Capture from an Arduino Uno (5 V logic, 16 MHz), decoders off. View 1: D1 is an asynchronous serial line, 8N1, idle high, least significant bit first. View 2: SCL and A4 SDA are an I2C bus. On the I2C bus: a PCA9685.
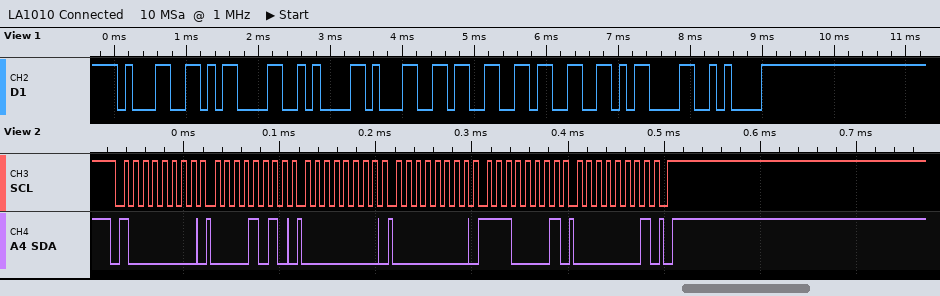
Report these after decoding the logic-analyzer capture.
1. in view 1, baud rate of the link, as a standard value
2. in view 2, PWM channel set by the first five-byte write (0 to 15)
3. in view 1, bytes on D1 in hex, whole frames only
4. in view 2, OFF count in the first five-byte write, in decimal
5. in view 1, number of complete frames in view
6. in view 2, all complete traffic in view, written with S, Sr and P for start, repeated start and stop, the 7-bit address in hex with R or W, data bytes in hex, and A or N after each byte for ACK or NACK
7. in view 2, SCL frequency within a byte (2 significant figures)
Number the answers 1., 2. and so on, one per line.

1. 9600 baud
2. 1
3. 31 0D 0A 31 33 33 0D 0A
4. 481
5. 8
6. S 40W A 0A A 00 A 00 A E1 A 01 A P
7. 100 kHz
